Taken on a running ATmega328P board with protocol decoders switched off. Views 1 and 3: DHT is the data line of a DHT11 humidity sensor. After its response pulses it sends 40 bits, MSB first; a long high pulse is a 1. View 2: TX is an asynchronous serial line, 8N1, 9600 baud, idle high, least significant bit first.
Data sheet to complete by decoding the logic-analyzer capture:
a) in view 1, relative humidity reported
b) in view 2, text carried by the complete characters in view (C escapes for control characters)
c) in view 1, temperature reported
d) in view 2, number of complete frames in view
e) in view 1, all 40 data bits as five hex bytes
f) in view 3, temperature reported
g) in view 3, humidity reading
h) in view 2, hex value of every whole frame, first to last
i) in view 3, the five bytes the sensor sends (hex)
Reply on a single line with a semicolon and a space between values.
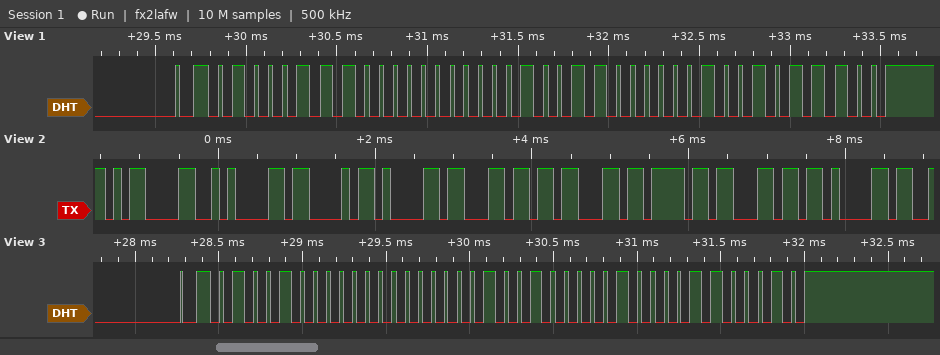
71 %; "\r\nCalcola"; 19.2 °C; 9; 47 00 13 02 5C; 18.8 °C; 72 %; 0D 0A 43 61 6C 63 6F 6C 61; 48 00 12 08 62
